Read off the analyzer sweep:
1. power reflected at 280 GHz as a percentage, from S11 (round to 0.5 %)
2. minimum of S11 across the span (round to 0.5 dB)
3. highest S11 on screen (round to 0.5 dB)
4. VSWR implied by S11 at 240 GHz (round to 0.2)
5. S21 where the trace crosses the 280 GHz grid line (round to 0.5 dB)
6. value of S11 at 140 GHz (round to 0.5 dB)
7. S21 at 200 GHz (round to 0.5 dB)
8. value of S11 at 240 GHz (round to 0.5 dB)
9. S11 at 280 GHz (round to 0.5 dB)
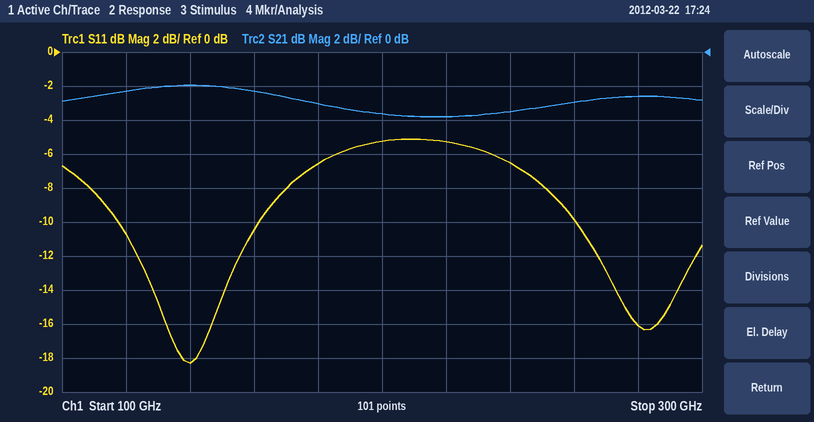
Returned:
2.5 %
-18.5 dB
-5.0 dB
2.8
-2.5 dB
-18.5 dB
-3.5 dB
-6.5 dB
-16.0 dB
